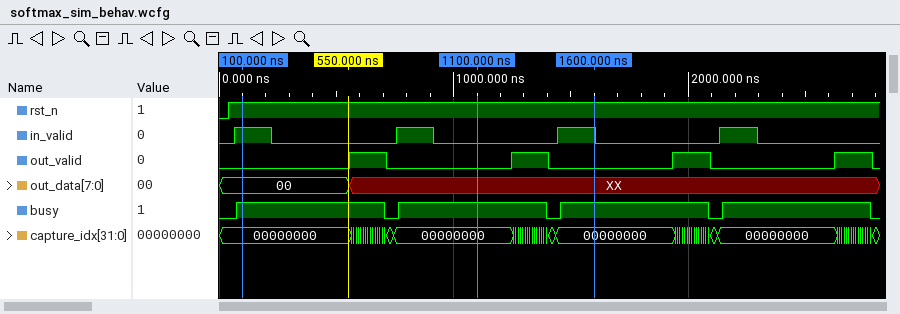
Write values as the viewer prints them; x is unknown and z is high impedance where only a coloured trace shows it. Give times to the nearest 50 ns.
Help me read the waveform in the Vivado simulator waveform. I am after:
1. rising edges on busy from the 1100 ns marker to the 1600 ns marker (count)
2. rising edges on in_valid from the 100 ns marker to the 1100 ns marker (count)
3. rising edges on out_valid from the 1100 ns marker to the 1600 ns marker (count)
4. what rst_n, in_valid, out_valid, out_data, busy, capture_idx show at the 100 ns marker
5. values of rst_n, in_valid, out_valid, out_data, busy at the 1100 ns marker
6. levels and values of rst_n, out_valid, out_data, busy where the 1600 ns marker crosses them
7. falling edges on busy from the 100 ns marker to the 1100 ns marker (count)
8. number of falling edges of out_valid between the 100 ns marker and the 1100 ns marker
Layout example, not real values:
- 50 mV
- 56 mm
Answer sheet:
- 1
- 1
- 1
- rst_n=1, in_valid=1, out_valid=0, out_data=00, busy=1, capture_idx=00000000
- rst_n=1, in_valid=0, out_valid=0, out_data=XX, busy=1
- rst_n=1, out_valid=0, out_data=XX, busy=1
- 1
- 1
